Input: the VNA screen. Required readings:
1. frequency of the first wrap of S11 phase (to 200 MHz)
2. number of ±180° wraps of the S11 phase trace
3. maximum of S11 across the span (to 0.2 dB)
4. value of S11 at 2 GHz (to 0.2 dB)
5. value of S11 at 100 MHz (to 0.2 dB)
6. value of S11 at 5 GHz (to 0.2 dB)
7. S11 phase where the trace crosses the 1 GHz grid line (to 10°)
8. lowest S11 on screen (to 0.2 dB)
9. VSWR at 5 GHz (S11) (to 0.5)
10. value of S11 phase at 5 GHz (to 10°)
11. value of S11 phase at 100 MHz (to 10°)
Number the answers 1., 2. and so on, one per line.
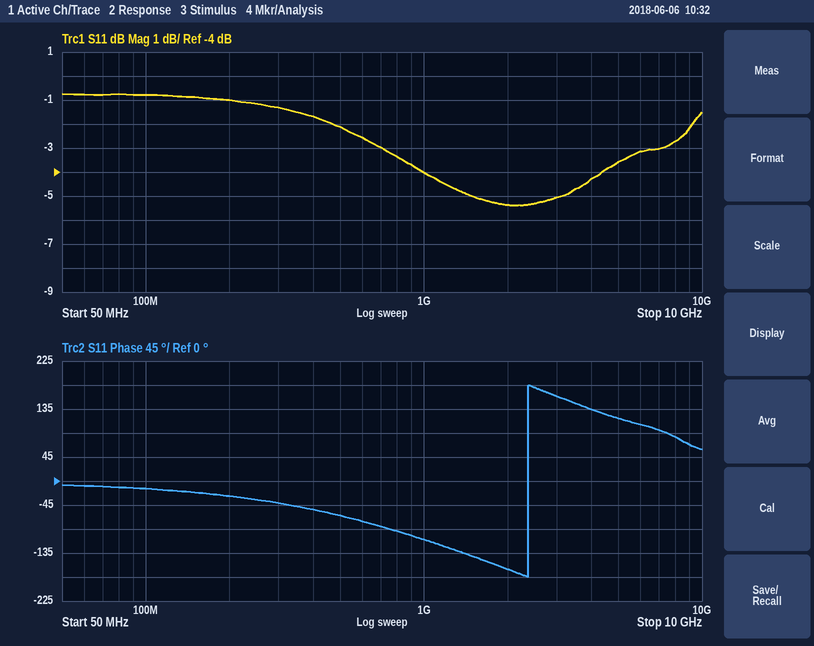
1. 2.4 GHz
2. 1
3. -0.8 dB
4. -5.4 dB
5. -0.8 dB
6. -3.6 dB
7. -110°
8. -5.4 dB
9. 5.0
10. 120°
11. -10°
